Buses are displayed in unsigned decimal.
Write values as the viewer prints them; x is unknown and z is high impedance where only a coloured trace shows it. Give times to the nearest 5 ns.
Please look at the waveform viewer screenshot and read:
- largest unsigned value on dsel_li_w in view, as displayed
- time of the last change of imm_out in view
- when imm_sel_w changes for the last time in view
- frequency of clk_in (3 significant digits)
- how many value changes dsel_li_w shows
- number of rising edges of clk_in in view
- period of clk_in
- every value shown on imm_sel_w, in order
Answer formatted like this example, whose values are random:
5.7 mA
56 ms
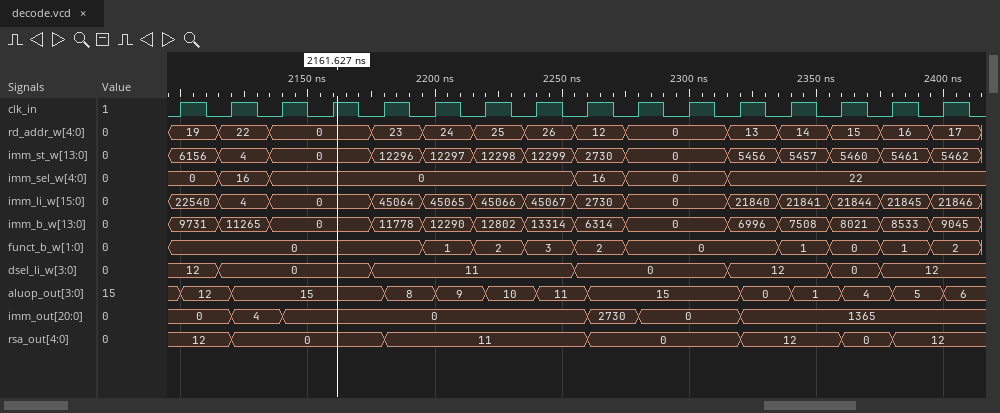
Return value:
12
2320 ns
2315 ns
50.0 MHz
6
16
20 ns
0, 16, 0, 16, 0, 22
